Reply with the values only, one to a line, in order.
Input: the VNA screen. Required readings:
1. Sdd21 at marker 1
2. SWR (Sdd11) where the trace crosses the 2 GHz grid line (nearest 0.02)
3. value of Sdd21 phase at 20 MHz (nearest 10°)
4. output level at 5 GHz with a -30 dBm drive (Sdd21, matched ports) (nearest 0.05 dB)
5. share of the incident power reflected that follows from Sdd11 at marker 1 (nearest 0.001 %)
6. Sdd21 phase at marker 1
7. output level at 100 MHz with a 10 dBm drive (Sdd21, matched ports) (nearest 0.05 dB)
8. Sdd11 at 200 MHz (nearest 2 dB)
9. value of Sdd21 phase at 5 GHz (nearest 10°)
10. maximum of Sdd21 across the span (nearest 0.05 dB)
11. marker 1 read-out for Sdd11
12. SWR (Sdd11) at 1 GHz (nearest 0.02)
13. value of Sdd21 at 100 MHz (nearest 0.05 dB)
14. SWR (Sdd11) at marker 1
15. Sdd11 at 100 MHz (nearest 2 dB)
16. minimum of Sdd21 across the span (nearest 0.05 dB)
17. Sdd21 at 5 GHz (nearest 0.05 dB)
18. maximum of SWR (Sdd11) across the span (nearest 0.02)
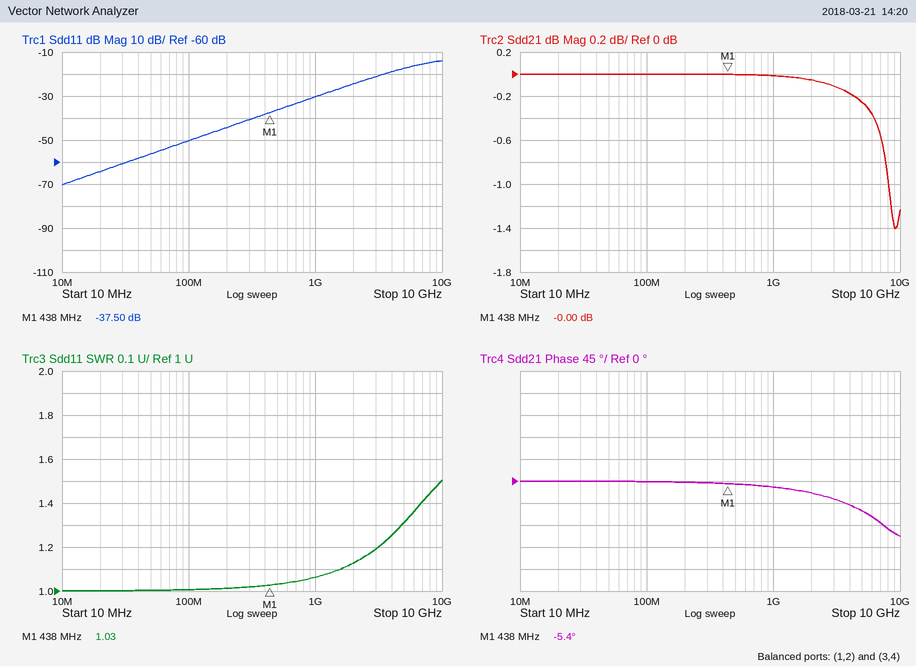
-0.00 dB
1.12
0°
-30.25 dBm
0.018 %
-5.4°
10.00 dBm
-44 dB
-60°
0.00 dB
-37.50 dB
1.06
0.00 dB
1.03
-50 dB
-1.40 dB
-0.25 dB
1.50
